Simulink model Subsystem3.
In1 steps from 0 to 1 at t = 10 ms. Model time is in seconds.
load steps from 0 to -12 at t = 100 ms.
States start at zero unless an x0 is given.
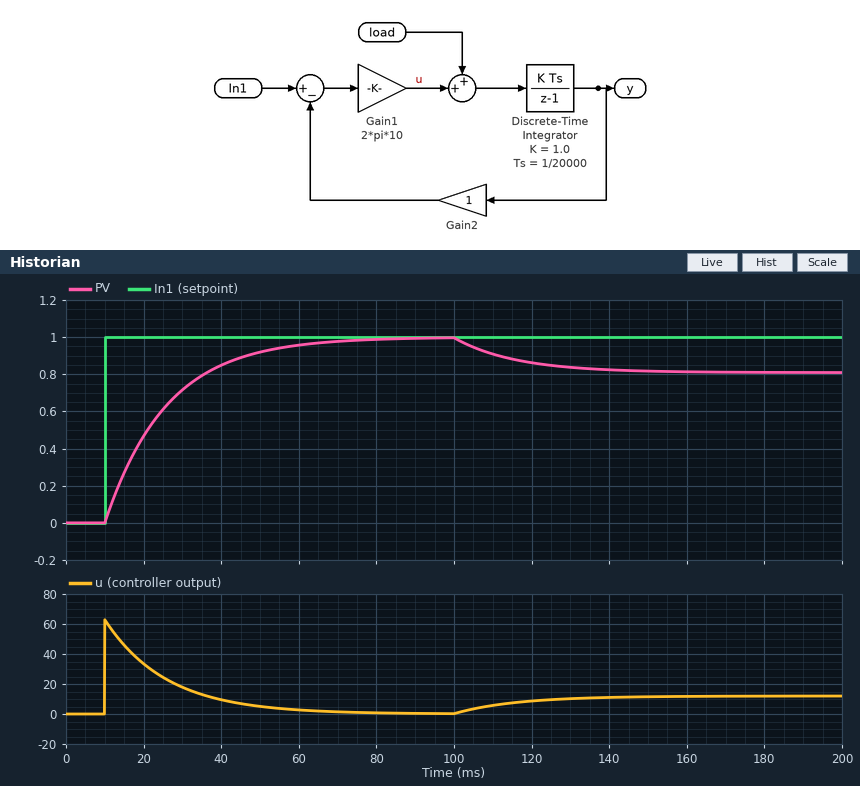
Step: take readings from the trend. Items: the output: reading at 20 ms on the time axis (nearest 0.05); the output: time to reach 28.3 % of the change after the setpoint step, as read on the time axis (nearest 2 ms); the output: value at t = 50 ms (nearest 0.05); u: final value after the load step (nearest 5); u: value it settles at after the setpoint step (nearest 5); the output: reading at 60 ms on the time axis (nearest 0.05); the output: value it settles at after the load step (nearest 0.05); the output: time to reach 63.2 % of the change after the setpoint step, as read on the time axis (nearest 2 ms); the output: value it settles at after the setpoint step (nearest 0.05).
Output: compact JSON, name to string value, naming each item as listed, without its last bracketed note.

{"the output: reading at 20 ms on the time axis": "0.45", "the output: time to reach 28.3 % of the change after the setpoint step, as read on the time axis": "16 ms", "the output: value at t = 50 ms": "0.90", "u: final value after the load step": "10", "u: value it settles at after the setpoint step": "0", "the output: reading at 60 ms on the time axis": "0.95", "the output: value it settles at after the load step": "0.80", "the output: time to reach 63.2 % of the change after the setpoint step, as read on the time axis": "26 ms", "the output: value it settles at after the setpoint step": "1.00"}
